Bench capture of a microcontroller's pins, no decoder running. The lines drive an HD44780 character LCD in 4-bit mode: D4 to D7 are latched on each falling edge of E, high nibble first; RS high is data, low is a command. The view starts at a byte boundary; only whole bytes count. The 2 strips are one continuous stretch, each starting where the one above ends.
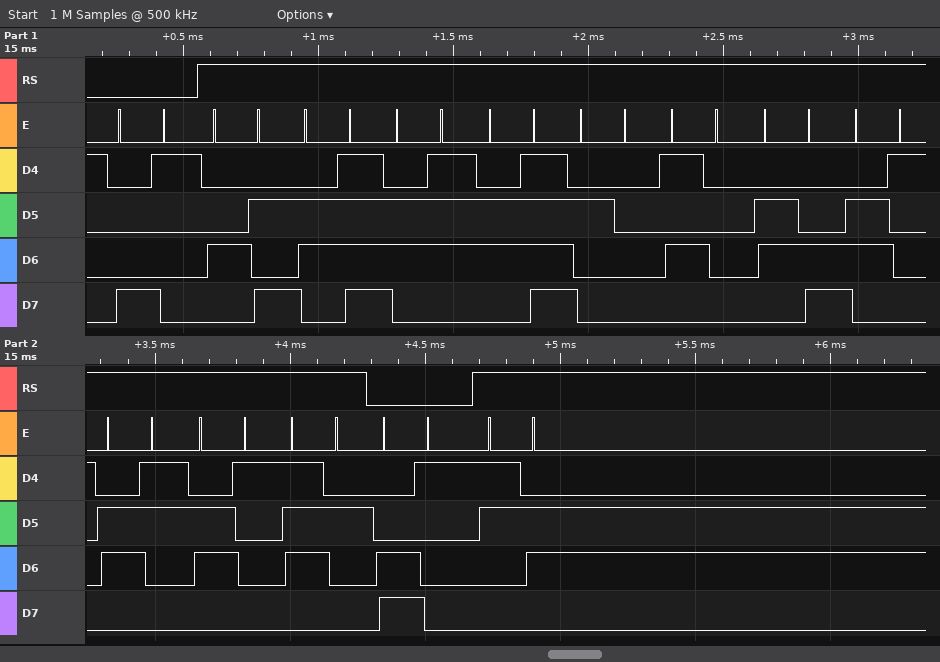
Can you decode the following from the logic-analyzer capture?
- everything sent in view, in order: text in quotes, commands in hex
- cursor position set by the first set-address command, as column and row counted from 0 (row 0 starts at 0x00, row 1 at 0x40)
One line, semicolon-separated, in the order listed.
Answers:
0x81 "Jogo Placar" 0xC1 "6"; column 1, row 0
